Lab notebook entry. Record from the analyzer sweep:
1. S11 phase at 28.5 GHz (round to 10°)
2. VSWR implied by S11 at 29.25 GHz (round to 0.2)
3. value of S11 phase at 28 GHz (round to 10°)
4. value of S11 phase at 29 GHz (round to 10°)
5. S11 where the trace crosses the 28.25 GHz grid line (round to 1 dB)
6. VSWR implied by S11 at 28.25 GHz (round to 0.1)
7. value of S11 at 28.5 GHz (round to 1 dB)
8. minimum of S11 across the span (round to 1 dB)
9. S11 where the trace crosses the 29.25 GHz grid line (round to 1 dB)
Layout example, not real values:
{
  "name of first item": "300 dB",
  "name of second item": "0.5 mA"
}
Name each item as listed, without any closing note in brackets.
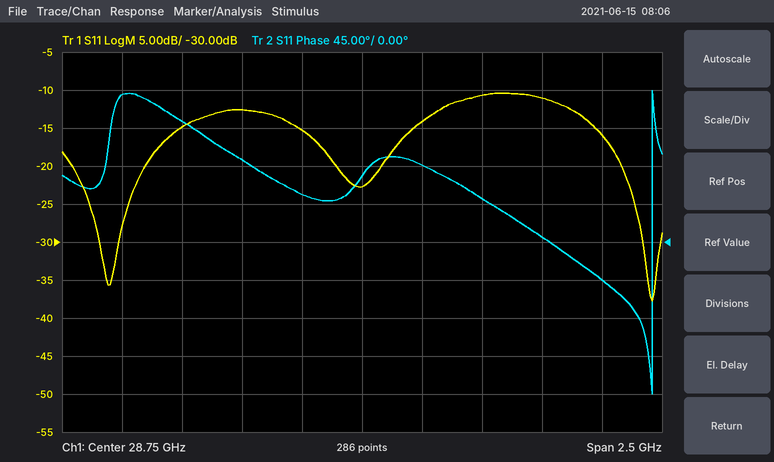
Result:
{
  "S11 phase at 28.5 GHz": "60°",
  "VSWR implied by S11 at 29.25 GHz": "1.8",
  "value of S11 phase at 28 GHz": "140°",
  "value of S11 phase at 29 GHz": "90°",
  "S11 where the trace crosses the 28.25 GHz grid line": "-13 dB",
  "VSWR implied by S11 at 28.25 GHz": "1.6",
  "value of S11 at 28.5 GHz": "-15 dB",
  "minimum of S11 across the span": "-38 dB",
  "S11 where the trace crosses the 29.25 GHz grid line": "-11 dB"
}
